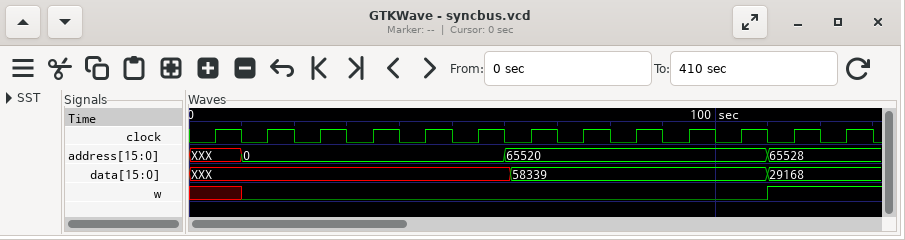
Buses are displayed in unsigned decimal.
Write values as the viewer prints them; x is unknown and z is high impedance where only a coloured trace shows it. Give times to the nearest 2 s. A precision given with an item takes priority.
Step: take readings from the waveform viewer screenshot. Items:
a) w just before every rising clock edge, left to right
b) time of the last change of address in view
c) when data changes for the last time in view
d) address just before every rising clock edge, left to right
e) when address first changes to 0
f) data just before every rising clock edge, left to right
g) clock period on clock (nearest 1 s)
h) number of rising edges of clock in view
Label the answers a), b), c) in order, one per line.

a) x 0 0 0 0 0 0 0 0 0 0 1 1
b) 110 s
c) 110 s
d) XXX, 0, 0, 0, 0, 0, 65520, 65520, 65520, 65520, 65520, 65528, 65528
e) 10 s
f) XXX, XXX, XXX, XXX, XXX, XXX, 58339, 58339, 58339, 58339, 58339, 29168, 29168
g) 10 s
h) 13
